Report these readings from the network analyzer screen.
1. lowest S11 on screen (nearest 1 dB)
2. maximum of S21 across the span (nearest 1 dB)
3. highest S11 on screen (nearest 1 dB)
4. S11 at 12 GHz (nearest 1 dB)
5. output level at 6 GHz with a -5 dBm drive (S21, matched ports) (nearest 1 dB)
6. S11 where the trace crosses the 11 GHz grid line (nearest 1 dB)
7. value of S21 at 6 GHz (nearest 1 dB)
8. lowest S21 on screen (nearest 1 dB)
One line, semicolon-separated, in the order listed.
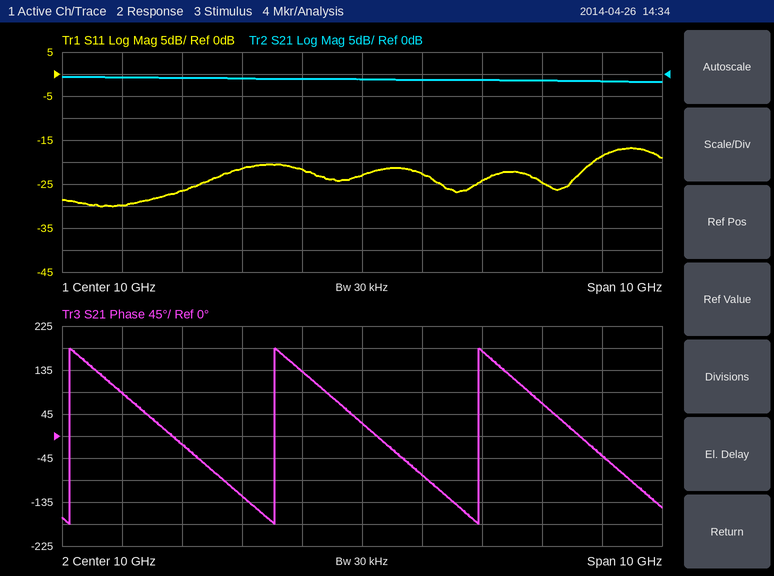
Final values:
-30 dB; -1 dB; -17 dB; -24 dB; -6 dBm; -23 dB; -1 dB; -2 dB
